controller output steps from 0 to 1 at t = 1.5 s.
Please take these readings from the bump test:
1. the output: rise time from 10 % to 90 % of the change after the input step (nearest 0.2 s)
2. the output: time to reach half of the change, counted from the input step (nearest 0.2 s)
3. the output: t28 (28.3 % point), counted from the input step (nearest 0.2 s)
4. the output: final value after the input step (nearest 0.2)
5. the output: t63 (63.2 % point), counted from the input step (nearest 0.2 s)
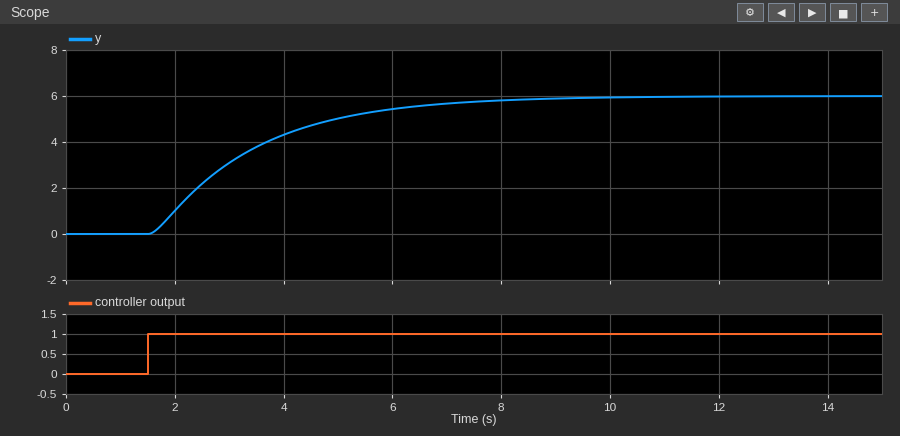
4.0 s
1.4 s
0.8 s
6.0
2.0 s
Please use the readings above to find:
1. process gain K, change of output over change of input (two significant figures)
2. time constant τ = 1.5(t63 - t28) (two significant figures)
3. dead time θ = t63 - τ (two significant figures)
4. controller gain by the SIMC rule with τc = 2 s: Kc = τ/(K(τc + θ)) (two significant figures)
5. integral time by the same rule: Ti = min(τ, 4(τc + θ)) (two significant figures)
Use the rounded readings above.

6.0
1.8 s
0.20 s
0.14
1.8 s
